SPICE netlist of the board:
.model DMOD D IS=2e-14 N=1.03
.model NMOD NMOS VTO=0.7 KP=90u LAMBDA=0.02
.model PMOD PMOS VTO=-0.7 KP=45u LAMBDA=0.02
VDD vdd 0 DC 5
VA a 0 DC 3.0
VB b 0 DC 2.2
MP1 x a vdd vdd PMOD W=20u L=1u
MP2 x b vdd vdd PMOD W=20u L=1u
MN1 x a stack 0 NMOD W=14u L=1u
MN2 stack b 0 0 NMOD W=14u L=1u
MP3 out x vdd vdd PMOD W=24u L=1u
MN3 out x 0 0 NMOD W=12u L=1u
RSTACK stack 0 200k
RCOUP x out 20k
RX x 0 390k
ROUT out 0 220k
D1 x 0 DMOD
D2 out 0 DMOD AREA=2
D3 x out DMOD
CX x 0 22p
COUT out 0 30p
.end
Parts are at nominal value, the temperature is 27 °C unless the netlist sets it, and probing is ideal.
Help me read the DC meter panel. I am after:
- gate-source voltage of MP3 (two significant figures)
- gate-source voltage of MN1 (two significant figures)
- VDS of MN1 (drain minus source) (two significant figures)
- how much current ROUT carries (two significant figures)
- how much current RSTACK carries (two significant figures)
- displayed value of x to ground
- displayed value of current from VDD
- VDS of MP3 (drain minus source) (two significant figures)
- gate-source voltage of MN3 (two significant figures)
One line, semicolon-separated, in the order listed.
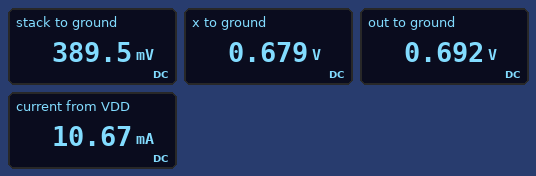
-4.3 V; 2.6 V; 290 mV; 3.1 µA; 1.9 µA; 0.679 V; 10.67 mA; -4.3 V; 680 mV
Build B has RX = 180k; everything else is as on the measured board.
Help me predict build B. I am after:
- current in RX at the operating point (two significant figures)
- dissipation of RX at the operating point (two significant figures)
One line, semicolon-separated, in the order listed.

3.8 µA; 2.6 µW
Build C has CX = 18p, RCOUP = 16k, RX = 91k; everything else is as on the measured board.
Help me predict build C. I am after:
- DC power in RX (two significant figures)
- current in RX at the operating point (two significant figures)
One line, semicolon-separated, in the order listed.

5.1 µW; 7.5 µA
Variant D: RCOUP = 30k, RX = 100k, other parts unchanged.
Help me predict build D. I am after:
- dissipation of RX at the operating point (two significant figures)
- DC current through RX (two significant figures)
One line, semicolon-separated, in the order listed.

4.6 µW; 6.8 µA
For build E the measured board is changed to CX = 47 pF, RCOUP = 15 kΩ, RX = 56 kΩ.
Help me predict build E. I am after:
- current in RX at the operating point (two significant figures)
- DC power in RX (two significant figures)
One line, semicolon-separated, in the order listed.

12 µA; 8.2 µW
